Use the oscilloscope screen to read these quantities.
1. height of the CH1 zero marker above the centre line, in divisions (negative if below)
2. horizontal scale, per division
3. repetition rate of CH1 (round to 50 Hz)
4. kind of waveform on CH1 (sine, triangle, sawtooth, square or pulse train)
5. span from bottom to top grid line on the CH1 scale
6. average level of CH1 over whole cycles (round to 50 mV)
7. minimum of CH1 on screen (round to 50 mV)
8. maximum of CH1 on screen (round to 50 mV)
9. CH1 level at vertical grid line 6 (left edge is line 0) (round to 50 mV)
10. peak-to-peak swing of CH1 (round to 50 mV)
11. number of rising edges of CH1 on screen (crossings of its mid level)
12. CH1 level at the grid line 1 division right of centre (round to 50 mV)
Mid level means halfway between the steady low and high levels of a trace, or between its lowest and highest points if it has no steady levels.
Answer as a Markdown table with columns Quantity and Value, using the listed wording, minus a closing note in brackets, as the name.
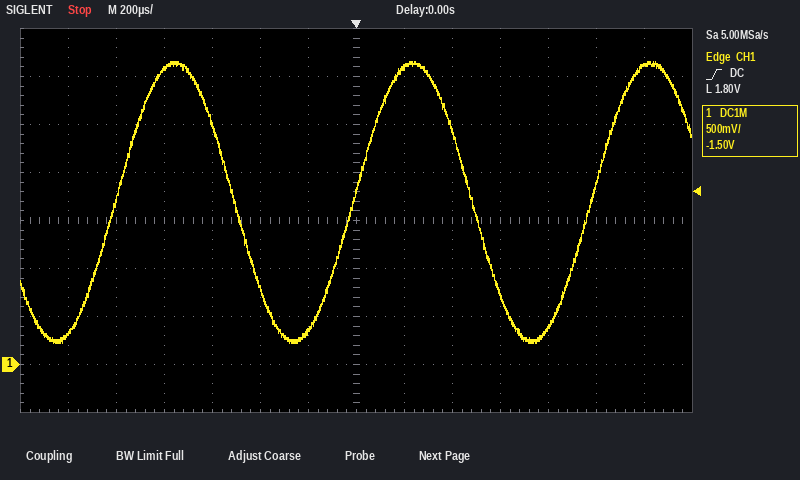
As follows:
| Quantity | Value |
|---|---|
| height of the CH1 zero marker above the centre line, in divisions | -3.0 div |
| horizontal scale, per division | 200 µs |
| repetition rate of CH1 | 1.00 kHz |
| kind of waveform on CH1 | sine |
| span from bottom to top grid line on the CH1 scale | 4 V |
| average level of CH1 over whole cycles | 1.70 V |
| minimum of CH1 on screen | 200 mV |
| maximum of CH1 on screen | 3.15 V |
| CH1 level at vertical grid line 6 (left edge is line 0) | 350 mV |
| peak-to-peak swing of CH1 | 2.95 V |
| number of rising edges of CH1 on screen | 3 |
| CH1 level at the grid line 1 division right of centre | 3.10 V |
